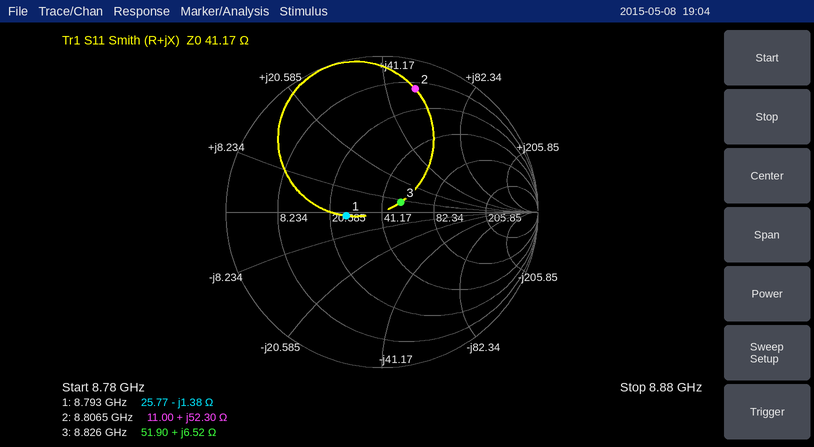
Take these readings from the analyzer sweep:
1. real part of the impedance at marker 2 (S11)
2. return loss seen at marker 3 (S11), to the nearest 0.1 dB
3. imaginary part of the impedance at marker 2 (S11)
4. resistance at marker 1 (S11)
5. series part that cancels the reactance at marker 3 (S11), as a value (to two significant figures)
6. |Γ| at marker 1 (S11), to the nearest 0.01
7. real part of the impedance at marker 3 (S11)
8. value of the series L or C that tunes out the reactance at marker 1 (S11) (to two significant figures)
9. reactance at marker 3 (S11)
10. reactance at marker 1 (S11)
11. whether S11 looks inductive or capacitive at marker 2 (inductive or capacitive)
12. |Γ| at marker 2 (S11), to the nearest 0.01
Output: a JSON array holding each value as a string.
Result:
["11.00 Ω", "17.4 dB", "+52.30 Ω", "25.77 Ω", "2.8 pF", "0.23", "51.90 Ω", "25 pH", "+6.52 Ω", "-1.38 Ω", "inductive", "0.82"]
